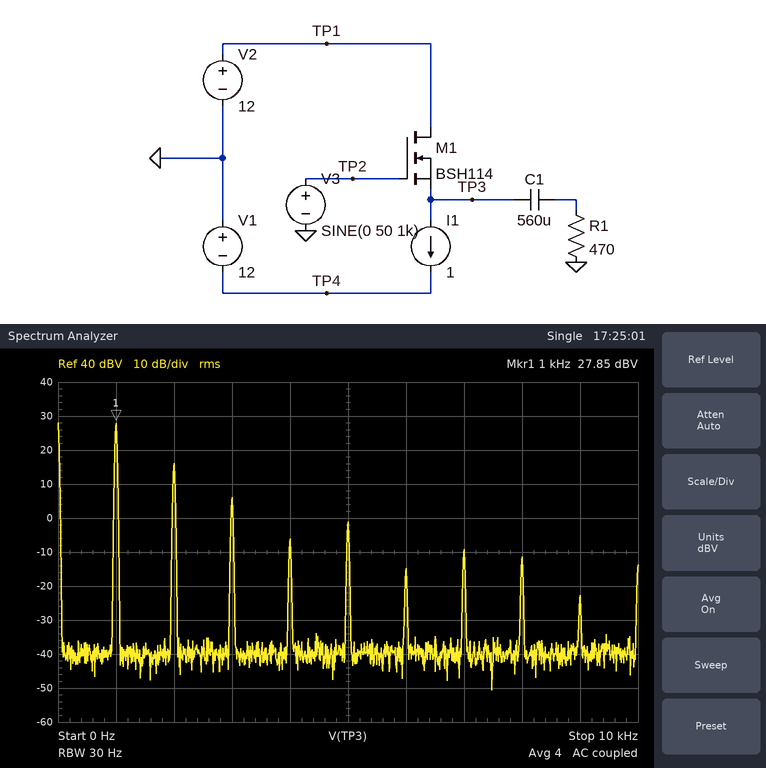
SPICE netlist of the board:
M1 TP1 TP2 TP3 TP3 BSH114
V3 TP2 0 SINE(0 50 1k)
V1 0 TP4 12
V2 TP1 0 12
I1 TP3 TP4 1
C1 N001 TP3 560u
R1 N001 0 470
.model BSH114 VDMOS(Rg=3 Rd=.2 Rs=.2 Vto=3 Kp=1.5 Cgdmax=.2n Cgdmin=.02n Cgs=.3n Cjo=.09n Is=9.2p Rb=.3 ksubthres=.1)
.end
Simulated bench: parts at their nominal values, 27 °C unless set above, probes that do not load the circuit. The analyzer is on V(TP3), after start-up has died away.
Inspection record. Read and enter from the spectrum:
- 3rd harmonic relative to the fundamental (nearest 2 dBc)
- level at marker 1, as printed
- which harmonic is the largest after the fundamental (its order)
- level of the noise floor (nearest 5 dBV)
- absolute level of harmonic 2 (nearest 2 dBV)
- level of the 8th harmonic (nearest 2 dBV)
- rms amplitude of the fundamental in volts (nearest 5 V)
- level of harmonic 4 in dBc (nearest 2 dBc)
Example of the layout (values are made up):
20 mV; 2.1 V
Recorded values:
-22 dBc; 27.85 dBV; 2; -40 dBV; 16 dBV; -12 dBV; 25 V; -34 dBc
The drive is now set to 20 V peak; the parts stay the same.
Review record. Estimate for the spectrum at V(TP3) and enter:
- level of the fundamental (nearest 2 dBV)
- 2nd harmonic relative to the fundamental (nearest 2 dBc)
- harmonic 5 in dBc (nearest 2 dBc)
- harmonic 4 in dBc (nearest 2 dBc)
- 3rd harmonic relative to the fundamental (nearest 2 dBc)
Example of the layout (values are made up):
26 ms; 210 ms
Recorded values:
22 dBV; -26 dBc; -36 dBc; -32 dBc; -28 dBc
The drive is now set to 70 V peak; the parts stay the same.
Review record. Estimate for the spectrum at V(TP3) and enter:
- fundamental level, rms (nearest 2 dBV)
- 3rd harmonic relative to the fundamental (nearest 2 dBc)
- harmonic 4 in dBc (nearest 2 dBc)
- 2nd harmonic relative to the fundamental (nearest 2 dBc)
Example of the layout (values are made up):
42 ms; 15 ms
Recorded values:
30 dBV; -24 dBc; -28 dBc; -10 dBc
